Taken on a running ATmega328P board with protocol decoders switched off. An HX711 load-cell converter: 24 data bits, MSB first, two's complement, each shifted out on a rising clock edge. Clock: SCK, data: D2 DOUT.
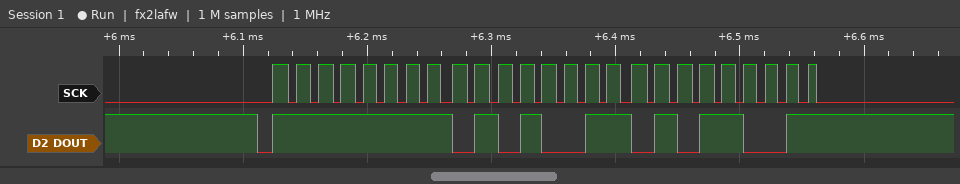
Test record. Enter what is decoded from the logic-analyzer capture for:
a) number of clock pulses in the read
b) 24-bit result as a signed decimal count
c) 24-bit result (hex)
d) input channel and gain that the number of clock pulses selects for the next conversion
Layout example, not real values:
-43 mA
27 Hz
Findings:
25
-44199
0xFF5359
channel A, gain 128
